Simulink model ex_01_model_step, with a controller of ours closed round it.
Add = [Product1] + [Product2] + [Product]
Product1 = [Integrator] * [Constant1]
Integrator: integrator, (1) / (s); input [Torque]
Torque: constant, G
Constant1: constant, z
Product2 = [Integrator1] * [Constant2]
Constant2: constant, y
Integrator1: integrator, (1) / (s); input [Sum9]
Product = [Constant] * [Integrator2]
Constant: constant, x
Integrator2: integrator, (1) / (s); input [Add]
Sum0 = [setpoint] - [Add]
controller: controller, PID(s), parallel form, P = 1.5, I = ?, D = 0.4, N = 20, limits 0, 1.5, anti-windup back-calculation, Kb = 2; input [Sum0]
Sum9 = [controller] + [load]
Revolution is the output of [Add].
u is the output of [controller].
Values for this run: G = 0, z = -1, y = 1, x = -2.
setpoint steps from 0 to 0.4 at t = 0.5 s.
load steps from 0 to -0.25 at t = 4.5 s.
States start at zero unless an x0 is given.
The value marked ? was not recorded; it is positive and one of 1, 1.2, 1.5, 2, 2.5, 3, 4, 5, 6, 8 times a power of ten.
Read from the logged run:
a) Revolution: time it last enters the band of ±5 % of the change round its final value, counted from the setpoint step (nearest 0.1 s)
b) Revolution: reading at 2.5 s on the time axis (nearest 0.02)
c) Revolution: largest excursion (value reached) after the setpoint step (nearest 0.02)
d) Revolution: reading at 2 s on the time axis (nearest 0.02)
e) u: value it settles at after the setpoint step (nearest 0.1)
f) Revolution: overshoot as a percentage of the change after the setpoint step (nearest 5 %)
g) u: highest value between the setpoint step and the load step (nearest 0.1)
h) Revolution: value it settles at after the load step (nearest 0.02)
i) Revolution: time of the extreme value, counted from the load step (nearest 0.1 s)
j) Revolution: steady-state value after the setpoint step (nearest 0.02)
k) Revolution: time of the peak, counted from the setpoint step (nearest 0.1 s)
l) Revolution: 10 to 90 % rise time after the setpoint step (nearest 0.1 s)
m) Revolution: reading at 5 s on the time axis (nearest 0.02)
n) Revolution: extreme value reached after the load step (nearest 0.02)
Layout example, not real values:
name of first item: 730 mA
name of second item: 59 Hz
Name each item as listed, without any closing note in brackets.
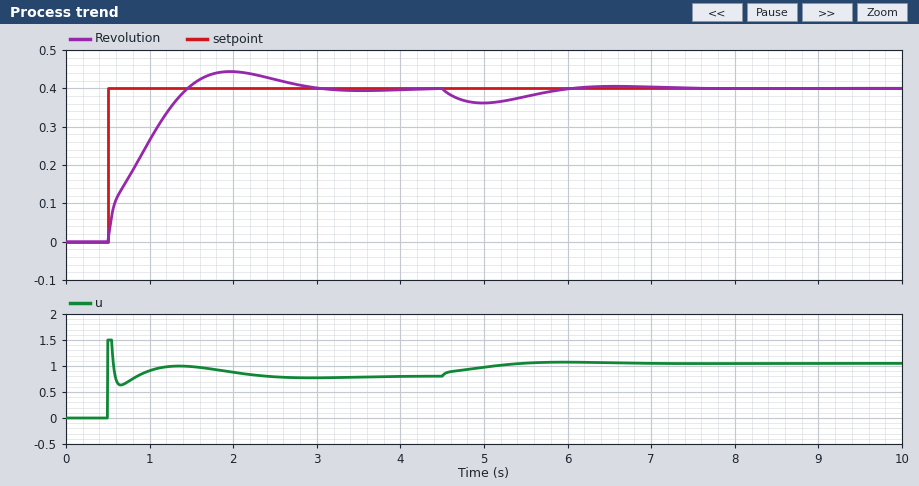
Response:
Revolution: time it last enters the band of ±5 % of the change round its final value, counted from the setpoint step: 2.1 s
Revolution: reading at 2.5 s on the time axis: 0.42
Revolution: largest excursion (value reached) after the setpoint step: 0.44
Revolution: reading at 2 s on the time axis: 0.44
u: value it settles at after the setpoint step: 0.8
Revolution: overshoot as a percentage of the change after the setpoint step: 10 %
u: highest value between the setpoint step and the load step: 1.5
Revolution: value it settles at after the load step: 0.40
Revolution: time of the extreme value, counted from the load step: 0.5 s
Revolution: steady-state value after the setpoint step: 0.40
Revolution: time of the peak, counted from the setpoint step: 1.5 s
Revolution: 10 to 90 % rise time after the setpoint step: 0.8 s
Revolution: reading at 5 s on the time axis: 0.36
Revolution: extreme value reached after the load step: 0.36
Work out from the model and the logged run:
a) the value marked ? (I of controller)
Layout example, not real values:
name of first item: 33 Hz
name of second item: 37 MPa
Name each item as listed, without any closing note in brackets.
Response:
the value marked ?: 8
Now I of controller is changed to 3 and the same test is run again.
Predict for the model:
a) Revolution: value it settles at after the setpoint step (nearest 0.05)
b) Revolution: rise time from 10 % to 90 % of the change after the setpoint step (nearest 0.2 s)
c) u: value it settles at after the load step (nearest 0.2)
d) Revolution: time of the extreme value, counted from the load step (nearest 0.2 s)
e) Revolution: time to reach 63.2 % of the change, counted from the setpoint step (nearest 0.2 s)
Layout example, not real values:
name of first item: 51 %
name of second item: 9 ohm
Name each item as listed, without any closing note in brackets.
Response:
Revolution: value it settles at after the setpoint step: 0.40
Revolution: rise time from 10 % to 90 % of the change after the setpoint step: 1.8 s
u: value it settles at after the load step: 1.0
Revolution: time of the extreme value, counted from the load step: 0.8 s
Revolution: time to reach 63.2 % of the change, counted from the setpoint step: 0.8 s
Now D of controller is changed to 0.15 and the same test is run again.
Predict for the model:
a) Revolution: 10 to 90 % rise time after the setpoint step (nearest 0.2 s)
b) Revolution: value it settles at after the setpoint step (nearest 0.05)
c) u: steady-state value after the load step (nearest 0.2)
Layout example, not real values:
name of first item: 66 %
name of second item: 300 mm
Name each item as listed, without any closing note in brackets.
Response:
Revolution: 10 to 90 % rise time after the setpoint step: 0.6 s
Revolution: value it settles at after the setpoint step: 0.40
u: steady-state value after the load step: 1.0
